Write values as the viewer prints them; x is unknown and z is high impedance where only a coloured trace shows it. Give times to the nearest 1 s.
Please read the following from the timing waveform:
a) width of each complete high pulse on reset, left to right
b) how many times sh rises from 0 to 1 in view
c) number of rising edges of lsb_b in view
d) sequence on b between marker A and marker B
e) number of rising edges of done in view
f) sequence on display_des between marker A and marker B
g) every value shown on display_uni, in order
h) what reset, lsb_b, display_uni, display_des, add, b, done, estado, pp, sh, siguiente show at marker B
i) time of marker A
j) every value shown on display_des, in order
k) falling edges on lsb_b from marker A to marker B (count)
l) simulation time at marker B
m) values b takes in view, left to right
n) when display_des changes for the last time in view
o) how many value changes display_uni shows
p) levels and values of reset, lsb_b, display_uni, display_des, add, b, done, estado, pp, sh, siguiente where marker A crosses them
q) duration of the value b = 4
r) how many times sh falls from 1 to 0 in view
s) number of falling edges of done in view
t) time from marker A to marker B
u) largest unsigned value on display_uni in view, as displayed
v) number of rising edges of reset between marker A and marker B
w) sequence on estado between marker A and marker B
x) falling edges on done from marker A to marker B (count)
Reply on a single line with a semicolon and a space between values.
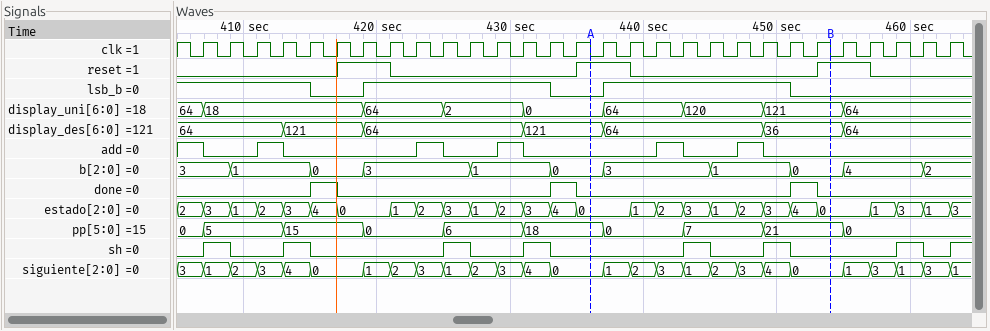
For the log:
4 s, 4 s, 4 s; 8; 2; 0, 3, 1, 0; 3; 121, 64, 36; 64, 18, 64, 2, 0, 64, 120, 121, 64; reset=1, lsb_b=0, display_uni=121, display_des=36, add=0, b=0, done=0, estado=0, pp=21, sh=0, siguiente=0; 436 s; 64, 121, 64, 121, 64, 36, 64; 1; 454 s; 3, 1, 0, 3, 1, 0, 3, 1, 0, 4, 2; 455 s; 8; reset=1, lsb_b=0, display_uni=0, display_des=121, add=0, b=0, done=0, estado=0, pp=18, sh=0, siguiente=0; 6 s; 7; 3; 18 s; 121; 1; 0, 1, 2, 3, 1, 2, 3, 4, 0; 1
